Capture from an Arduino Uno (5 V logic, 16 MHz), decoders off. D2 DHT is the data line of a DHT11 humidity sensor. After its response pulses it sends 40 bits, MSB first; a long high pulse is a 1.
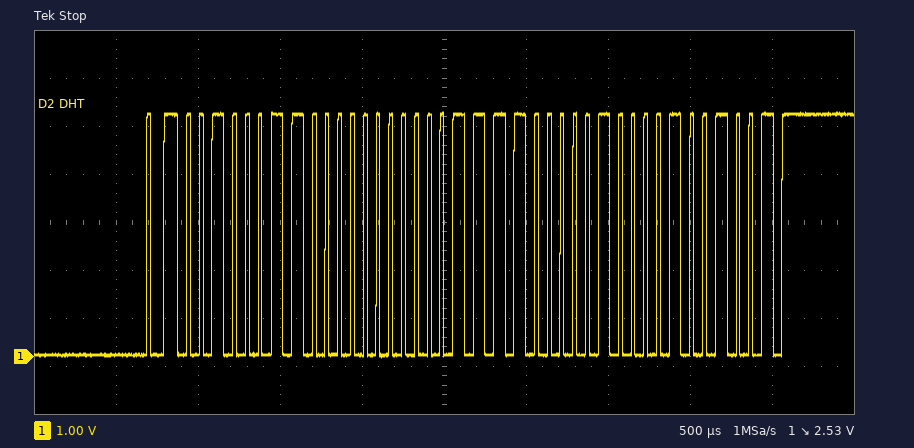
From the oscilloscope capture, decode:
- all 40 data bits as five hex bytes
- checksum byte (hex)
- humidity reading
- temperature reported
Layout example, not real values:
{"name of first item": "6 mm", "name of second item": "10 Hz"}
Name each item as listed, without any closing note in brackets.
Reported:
{"all 40 data bits as five hex bytes": "23 00 1E 08 49", "checksum byte": "0x49", "humidity reading": "35 %", "temperature reported": "30.8 °C"}
